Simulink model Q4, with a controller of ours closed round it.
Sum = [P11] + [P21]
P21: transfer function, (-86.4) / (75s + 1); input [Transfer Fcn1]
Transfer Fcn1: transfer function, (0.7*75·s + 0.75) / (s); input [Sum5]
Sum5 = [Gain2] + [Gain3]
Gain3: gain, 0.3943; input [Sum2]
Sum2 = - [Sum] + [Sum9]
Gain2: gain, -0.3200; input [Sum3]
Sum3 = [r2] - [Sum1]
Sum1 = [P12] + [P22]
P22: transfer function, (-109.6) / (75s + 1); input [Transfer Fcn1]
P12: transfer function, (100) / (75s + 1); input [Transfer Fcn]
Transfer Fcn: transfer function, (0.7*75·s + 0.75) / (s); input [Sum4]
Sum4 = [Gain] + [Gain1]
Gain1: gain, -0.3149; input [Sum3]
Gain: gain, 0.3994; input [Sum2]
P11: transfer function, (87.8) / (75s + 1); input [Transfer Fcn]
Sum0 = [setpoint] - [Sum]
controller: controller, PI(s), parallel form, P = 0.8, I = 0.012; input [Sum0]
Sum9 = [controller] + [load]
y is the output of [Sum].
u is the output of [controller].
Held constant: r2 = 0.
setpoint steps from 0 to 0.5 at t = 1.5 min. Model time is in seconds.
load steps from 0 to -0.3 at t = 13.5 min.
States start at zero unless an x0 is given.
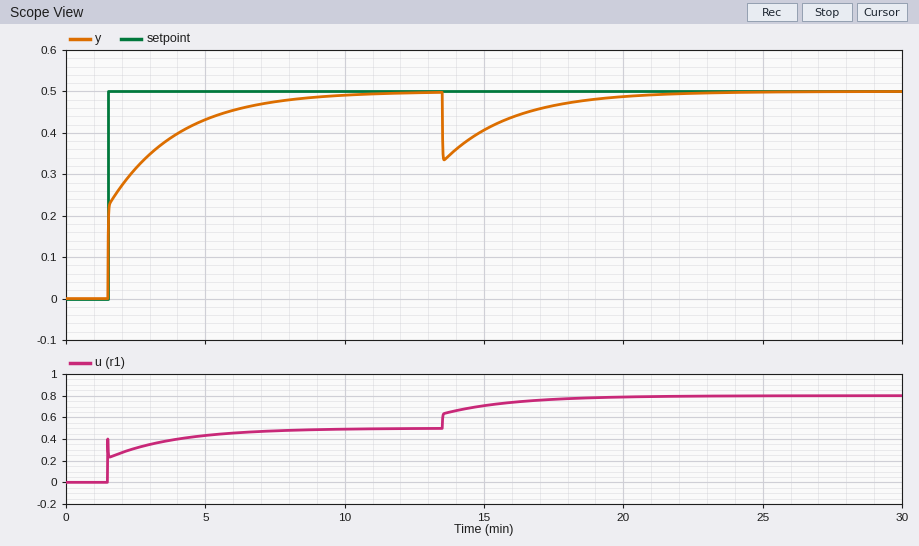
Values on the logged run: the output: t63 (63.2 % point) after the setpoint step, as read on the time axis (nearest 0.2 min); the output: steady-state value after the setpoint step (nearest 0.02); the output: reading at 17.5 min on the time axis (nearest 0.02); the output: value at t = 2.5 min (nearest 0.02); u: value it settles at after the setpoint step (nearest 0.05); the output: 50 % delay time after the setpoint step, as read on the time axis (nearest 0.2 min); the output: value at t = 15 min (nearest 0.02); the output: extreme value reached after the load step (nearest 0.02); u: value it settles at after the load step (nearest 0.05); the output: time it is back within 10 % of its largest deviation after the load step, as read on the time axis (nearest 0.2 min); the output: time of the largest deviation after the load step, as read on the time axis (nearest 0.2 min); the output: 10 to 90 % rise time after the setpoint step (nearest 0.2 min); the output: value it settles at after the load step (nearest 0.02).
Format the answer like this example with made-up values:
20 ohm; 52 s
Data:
2.6 min; 0.50; 0.46; 0.32; 0.50; 1.8 min; 0.40; 0.34; 0.80; 19.4 min; 13.6 min; 4.2 min; 0.50
